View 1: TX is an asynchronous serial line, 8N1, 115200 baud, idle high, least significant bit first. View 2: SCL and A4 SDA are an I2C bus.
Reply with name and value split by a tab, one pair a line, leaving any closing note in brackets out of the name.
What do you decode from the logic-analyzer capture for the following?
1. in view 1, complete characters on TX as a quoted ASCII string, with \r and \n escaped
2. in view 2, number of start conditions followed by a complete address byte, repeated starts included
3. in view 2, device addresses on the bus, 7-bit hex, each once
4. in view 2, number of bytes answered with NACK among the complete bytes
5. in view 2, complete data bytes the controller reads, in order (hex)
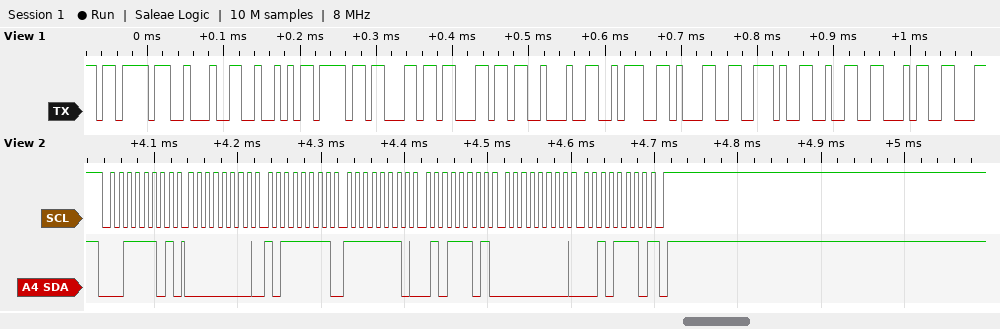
in view 1, complete characters on TX as a quoted ASCII string, with \r and \n escaped	"{\"Roll\":1.24"
in view 2, number of start conditions followed by a complete address byte, repeated starts included	1
in view 2, device addresses on the bus, 7-bit hex, each once	0x1E
in view 2, number of bytes answered with NACK among the complete bytes	1
in view 2, complete data bytes the controller reads, in order	00 BF FE 5D 00 2E
